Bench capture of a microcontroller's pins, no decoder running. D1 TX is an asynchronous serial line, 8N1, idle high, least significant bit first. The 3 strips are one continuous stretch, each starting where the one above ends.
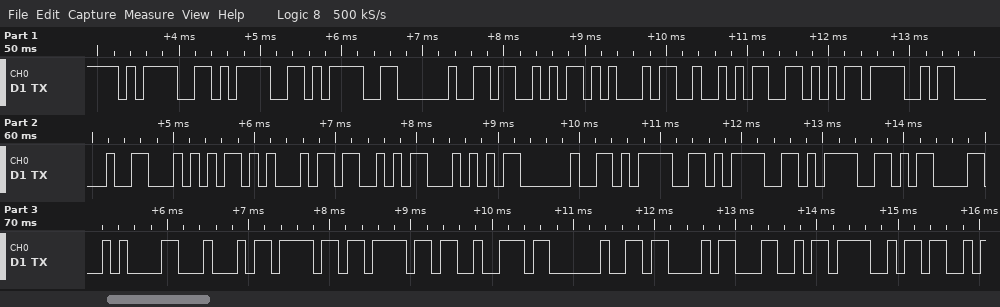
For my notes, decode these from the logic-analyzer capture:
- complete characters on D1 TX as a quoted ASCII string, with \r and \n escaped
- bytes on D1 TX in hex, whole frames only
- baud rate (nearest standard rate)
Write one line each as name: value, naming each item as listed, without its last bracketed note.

complete characters on D1 TX as a quoted ASCII string, with \r and \n escaped: "=== SERVO TEST ===\r\nDoor CLO"
bytes on D1 TX in hex, whole frames only: 3D 3D 3D 20 53 45 52 56 4F 20 54 45 53 54 20 3D 3D 3D 0D 0A 44 6F 6F 72 20 43 4C 4F
baud rate: 9600 baud
